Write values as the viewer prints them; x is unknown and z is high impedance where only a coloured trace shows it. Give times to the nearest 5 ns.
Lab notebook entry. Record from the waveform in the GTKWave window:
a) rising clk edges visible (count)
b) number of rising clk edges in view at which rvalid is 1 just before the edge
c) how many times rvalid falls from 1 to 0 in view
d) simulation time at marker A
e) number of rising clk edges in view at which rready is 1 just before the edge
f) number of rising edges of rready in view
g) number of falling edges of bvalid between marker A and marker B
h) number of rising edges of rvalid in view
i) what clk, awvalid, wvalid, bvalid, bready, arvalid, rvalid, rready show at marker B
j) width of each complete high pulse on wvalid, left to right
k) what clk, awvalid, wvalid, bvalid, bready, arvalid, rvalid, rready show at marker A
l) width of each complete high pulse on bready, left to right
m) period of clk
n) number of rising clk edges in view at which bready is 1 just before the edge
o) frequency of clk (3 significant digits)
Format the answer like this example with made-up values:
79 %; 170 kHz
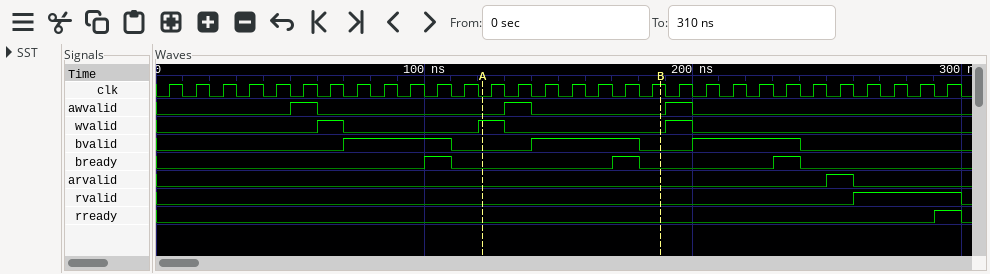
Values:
30; 4; 1; 120 ns; 1; 1; 1; 1; clk=1, awvalid=0, wvalid=0, bvalid=0, bready=0, arvalid=0, rvalid=0, rready=0; 10 ns, 10 ns, 10 ns; clk=0, awvalid=0, wvalid=1, bvalid=0, bready=0, arvalid=0, rvalid=0, rready=0; 10 ns, 10 ns, 10 ns; 10 ns; 3; 100 MHz
